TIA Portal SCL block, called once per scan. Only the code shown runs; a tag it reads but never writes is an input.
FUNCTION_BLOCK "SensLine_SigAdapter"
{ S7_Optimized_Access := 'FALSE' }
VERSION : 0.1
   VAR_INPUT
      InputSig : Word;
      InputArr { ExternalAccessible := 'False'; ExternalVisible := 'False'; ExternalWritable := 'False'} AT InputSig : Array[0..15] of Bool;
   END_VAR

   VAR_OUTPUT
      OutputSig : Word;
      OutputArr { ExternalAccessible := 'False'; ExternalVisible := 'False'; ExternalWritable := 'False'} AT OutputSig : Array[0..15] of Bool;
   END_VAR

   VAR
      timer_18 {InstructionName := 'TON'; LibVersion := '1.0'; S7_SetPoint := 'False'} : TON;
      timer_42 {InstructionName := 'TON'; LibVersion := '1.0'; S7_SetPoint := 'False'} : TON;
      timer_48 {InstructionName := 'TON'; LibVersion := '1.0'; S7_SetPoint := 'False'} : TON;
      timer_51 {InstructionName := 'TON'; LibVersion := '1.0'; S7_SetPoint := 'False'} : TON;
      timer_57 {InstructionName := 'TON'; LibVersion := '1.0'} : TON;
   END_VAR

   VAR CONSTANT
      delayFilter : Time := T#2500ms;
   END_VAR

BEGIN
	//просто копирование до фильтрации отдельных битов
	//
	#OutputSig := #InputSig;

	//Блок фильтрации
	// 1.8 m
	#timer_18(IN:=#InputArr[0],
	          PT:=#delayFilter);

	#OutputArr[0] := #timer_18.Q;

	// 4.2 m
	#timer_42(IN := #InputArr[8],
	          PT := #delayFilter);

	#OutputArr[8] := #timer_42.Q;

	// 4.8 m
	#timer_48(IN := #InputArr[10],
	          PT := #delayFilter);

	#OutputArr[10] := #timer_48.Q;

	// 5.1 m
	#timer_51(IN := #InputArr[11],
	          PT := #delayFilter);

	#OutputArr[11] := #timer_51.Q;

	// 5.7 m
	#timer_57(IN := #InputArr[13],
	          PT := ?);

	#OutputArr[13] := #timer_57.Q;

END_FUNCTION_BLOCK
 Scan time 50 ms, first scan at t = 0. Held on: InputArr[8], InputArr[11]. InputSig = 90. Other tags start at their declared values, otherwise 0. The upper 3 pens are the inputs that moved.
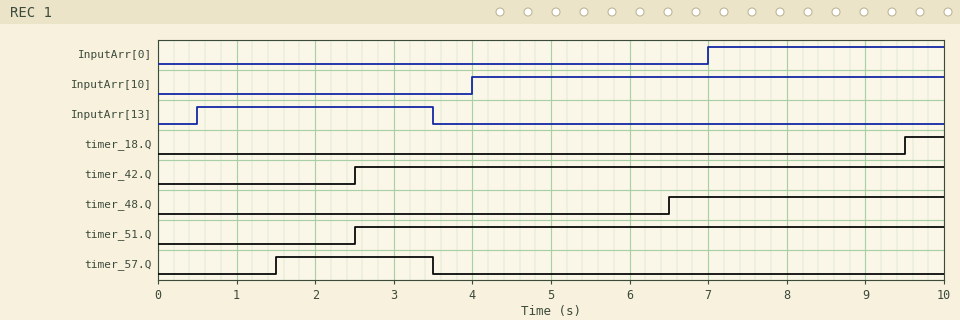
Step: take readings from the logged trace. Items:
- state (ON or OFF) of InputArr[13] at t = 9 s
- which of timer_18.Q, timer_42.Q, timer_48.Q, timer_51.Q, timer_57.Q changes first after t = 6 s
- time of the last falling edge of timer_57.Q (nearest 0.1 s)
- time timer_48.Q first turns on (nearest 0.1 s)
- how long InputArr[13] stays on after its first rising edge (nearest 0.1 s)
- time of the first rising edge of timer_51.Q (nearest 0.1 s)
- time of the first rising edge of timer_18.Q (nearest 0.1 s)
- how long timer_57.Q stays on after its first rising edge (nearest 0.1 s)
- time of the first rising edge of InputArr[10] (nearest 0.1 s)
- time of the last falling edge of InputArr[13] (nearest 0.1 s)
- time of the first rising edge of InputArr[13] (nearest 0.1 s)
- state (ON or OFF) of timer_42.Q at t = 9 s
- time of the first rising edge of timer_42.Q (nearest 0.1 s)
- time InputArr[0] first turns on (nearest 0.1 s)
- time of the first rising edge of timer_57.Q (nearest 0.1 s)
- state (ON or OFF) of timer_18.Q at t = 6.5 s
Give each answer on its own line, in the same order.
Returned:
OFF
timer_48.Q
3.5 s
6.5 s
3.0 s
2.5 s
9.5 s
2.0 s
4.0 s
3.5 s
0.5 s
ON
2.5 s
7.0 s
1.5 s
OFF
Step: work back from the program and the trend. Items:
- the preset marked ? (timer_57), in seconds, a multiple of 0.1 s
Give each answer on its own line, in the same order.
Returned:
1.0 s
